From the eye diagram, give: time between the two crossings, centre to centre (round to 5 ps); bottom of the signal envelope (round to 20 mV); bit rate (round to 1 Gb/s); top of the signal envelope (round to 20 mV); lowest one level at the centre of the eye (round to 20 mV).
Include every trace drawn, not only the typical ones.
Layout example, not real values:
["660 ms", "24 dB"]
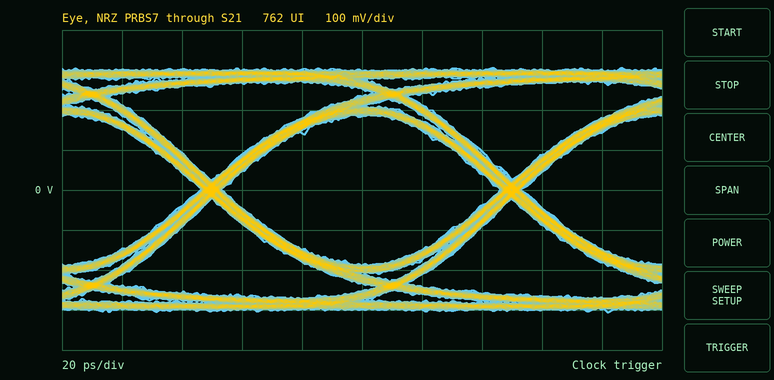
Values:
["100 ps", "-300 mV", "10 Gb/s", "300 mV", "180 mV"]
